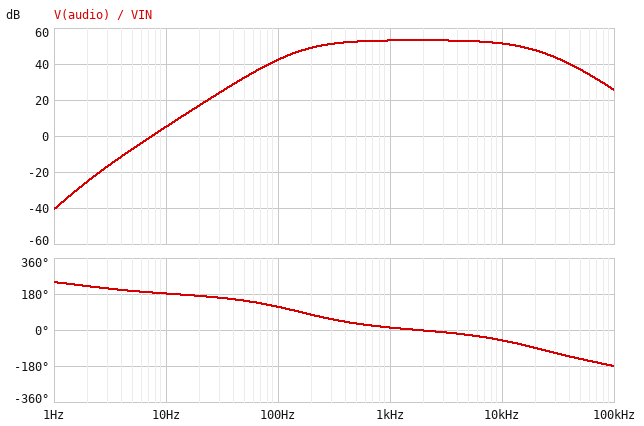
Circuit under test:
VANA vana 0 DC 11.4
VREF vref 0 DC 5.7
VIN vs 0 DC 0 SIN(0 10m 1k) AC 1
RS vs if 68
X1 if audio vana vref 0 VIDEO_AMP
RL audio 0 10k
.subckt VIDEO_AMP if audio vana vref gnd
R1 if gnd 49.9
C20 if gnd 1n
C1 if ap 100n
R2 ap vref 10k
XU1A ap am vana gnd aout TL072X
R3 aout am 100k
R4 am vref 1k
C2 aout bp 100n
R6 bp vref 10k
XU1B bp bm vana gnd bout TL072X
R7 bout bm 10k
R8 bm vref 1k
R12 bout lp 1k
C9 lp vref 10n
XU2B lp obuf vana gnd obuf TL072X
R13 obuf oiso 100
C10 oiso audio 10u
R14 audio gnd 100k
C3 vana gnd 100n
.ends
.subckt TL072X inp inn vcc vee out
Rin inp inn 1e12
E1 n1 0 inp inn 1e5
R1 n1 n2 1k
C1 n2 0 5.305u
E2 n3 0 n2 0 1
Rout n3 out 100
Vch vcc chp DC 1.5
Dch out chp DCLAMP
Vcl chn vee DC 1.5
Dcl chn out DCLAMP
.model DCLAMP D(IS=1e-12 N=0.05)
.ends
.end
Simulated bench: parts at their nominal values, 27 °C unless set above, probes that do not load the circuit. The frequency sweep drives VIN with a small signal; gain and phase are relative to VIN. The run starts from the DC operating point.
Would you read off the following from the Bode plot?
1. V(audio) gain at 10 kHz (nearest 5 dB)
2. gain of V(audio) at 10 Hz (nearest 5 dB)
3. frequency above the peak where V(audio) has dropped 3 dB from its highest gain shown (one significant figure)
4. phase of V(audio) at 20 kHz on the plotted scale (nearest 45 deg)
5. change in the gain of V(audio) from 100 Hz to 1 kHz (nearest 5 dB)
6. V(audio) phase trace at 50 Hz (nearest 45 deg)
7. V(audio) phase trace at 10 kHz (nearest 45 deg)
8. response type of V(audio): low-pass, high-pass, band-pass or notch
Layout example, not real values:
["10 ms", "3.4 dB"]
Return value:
["50 dB", "5 dB", "10 kHz", "-90 deg", "10 dB", "135 deg", "-45 deg", "band-pass"]
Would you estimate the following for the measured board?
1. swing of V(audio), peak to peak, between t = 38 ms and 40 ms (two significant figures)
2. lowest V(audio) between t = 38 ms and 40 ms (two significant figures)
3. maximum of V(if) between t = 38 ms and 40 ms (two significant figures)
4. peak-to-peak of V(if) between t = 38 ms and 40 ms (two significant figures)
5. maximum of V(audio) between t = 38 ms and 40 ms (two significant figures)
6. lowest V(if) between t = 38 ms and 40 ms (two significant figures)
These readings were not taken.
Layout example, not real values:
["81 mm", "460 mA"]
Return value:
["8.4 V", "-4.2 V", "4.2 mV", "8.4 mV", "4.2 V", "-4.2 mV"]
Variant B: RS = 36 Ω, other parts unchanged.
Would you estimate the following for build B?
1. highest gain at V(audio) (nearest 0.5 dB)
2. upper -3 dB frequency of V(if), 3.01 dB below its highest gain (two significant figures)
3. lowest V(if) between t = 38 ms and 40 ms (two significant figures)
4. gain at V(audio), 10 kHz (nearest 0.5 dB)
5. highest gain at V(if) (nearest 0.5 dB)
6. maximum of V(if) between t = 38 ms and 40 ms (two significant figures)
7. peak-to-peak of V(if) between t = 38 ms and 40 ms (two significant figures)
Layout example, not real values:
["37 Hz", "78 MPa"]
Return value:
["56.0 dB", "7.6 MHz", "-5.8 mV", "54.0 dB", "-4.5 dB", "5.8 mV", "12 mV"]
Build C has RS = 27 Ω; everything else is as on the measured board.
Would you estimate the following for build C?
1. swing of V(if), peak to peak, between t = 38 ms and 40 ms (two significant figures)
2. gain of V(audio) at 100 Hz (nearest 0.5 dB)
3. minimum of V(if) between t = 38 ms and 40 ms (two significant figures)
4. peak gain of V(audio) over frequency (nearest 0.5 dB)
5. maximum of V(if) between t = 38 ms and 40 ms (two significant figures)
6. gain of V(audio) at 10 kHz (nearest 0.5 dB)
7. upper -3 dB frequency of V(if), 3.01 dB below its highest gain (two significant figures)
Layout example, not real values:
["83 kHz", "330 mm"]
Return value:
["13 mV", "46.0 dB", "-6.5 mV", "57.0 dB", "6.5 mV", "55.0 dB", "9.1 MHz"]
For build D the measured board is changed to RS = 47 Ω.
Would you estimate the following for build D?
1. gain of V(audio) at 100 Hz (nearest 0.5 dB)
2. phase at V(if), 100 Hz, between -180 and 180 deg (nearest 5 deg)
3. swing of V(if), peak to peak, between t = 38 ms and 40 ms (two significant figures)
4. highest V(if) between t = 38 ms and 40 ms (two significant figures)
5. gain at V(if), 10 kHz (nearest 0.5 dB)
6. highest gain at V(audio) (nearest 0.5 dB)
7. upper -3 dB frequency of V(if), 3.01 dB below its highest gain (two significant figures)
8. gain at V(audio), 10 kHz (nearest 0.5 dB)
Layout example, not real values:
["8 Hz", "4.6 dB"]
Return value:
["44.0 dB", "0 deg", "10 mV", "5.1 mV", "-6.0 dB", "55.0 dB", "6.6 MHz", "53.0 dB"]
